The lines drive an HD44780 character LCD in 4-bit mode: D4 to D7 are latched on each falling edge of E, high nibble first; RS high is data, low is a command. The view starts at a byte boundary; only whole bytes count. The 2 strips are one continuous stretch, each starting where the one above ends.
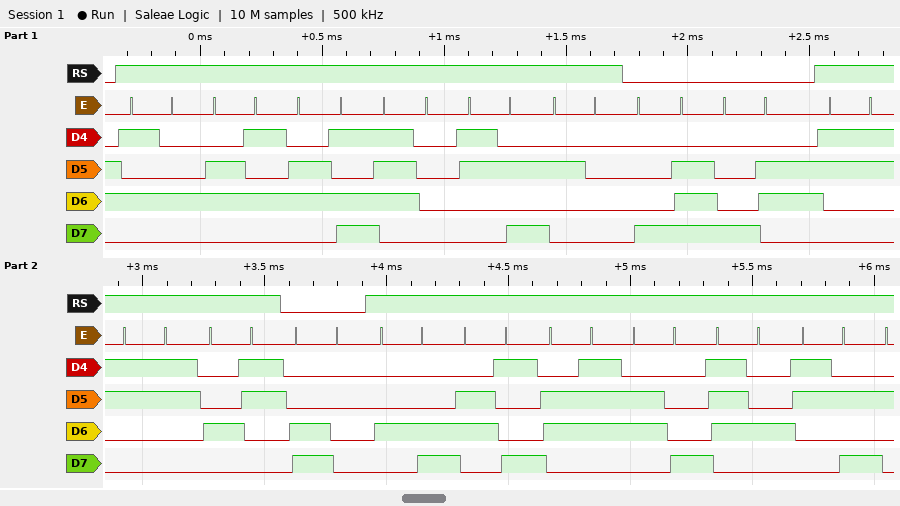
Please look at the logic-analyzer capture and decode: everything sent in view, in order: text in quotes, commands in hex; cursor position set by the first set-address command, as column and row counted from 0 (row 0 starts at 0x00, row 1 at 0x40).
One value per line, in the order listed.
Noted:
"Temp: " 0x8E 0x86 "33C" 0xC0 "Light:"
column 14, row 0
